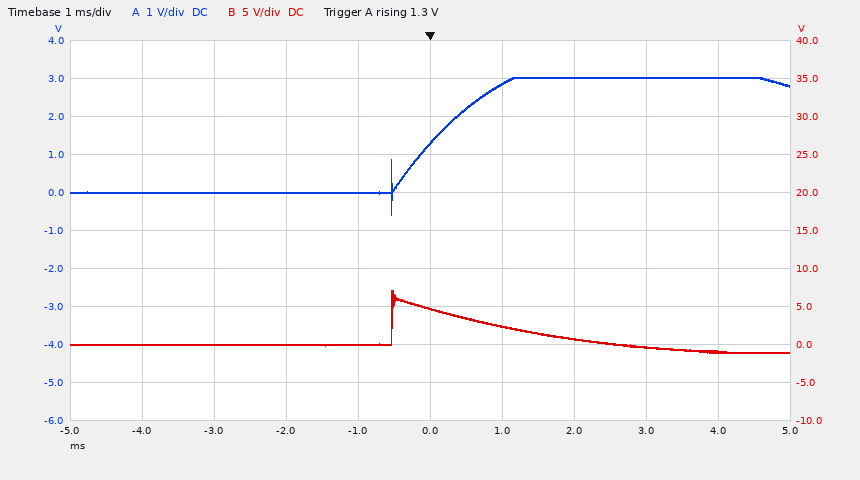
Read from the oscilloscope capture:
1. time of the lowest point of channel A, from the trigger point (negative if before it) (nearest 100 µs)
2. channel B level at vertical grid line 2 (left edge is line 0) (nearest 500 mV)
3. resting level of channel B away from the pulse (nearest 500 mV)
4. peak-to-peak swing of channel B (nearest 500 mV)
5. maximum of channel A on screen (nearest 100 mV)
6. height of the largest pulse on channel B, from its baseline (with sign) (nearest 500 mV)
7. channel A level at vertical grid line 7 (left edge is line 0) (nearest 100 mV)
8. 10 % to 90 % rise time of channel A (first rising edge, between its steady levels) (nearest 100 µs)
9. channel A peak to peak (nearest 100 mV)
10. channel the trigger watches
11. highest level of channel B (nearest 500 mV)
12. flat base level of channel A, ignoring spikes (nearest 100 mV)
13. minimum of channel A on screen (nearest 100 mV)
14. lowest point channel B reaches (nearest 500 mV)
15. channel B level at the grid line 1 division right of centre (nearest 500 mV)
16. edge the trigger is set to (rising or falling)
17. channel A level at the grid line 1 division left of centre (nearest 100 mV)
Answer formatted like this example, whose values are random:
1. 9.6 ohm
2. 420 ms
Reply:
1. -500 µs
2. 0.0 V
3. 0.0 V
4. 8.0 V
5. 3.0 V
6. +7.0 V
7. 3.0 V
8. 1.3 ms
9. 3.6 V
10. channel A
11. 7.0 V
12. 0.0 V
13. -600 mV
14. -1.0 V
15. 2.5 V
16. rising
17. 0.0 V
